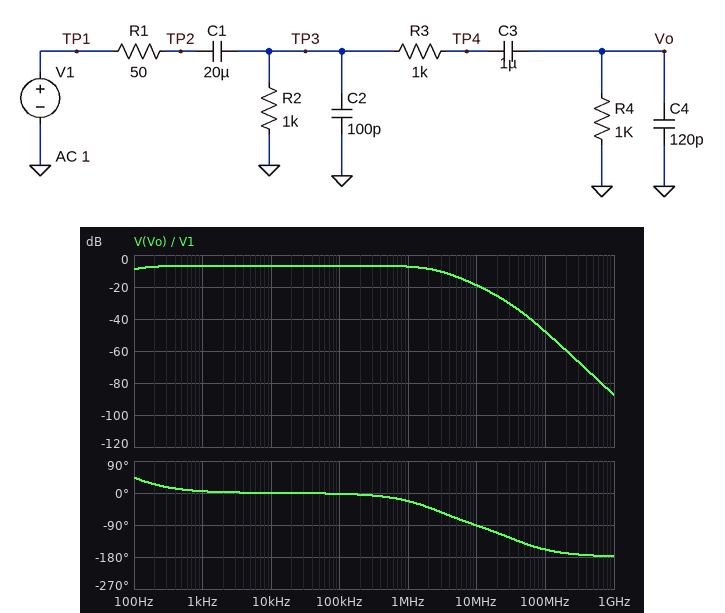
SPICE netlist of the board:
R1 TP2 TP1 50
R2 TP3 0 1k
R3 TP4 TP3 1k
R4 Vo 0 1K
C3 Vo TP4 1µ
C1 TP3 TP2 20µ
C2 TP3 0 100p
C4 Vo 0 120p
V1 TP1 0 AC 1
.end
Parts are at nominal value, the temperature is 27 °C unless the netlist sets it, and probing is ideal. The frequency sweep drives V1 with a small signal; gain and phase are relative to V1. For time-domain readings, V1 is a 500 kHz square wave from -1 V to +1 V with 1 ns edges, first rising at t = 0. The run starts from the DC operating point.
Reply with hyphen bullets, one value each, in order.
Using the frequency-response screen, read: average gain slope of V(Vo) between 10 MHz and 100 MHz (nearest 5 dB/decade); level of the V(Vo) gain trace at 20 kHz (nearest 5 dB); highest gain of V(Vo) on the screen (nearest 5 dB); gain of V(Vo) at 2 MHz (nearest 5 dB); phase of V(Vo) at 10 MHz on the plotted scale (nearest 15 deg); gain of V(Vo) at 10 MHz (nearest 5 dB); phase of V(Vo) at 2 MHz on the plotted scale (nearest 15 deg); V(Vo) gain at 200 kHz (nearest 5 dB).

- -30 dB/decade
- -5 dB
- -5 dB
- -10 dB
- -90 deg
- -20 dB
- -45 deg
- -5 dB
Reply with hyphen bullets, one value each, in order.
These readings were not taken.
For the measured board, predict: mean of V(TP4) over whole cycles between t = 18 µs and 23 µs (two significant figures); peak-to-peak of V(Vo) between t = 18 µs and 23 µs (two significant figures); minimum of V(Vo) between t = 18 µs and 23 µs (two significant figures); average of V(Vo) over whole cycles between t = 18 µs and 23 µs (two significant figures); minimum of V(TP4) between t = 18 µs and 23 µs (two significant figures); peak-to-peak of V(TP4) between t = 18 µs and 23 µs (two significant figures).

- 470 mV
- 930 mV
- -5.7 mV
- 460 mV
- 3.7 mV
- 930 mV
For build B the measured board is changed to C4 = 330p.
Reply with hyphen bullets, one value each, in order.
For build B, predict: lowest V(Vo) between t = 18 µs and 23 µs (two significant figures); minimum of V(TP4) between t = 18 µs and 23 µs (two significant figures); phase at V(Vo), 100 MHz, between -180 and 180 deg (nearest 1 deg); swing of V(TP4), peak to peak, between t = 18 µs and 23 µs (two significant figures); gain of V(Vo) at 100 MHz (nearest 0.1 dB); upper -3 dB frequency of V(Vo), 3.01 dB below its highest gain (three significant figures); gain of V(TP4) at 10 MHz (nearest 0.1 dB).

- -3.1 mV
- 6.2 mV
- -160 deg
- 930 mV
- -56.8 dB
- 942 kHz
- -27.5 dB
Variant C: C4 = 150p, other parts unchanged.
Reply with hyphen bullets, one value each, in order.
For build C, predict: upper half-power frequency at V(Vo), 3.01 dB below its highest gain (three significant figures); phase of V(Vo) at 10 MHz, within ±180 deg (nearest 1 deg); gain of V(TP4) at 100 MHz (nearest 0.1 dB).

- 2.06 MHz
- -94 deg
- -49.9 dB
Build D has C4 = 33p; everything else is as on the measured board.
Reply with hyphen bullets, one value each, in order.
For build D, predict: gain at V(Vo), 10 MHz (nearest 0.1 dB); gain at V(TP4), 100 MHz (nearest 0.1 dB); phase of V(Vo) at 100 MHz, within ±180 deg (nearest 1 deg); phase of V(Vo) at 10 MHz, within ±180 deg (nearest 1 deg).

- -10.3 dB
- -36.8 dB
- -155 deg
- -63 deg
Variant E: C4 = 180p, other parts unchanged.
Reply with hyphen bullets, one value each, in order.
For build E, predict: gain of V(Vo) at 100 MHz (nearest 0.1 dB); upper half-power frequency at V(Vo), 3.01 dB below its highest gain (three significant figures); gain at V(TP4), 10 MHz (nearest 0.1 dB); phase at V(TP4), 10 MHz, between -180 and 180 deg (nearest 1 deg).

- -51.5 dB
- 1.72 MHz
- -22.4 dB
- -96 deg
